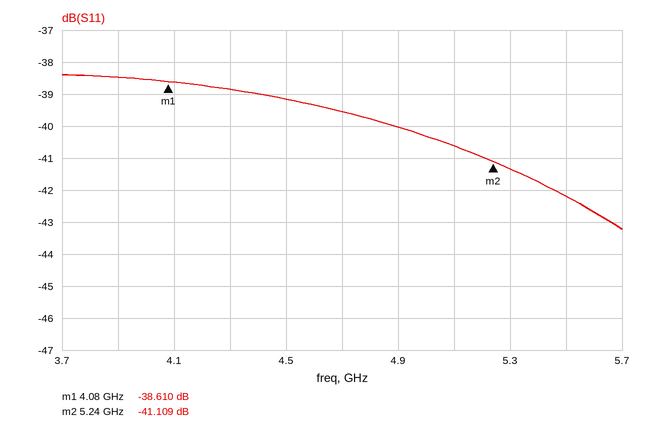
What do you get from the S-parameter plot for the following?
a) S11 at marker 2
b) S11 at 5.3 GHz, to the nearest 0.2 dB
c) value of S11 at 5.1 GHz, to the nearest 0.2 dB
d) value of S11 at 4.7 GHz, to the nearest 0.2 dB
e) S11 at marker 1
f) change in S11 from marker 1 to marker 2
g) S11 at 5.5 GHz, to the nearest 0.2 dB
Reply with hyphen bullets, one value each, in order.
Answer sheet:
- -41.109 dB
- -41.4 dB
- -40.6 dB
- -39.6 dB
- -38.610 dB
- -2.499 dB
- -42.2 dB
